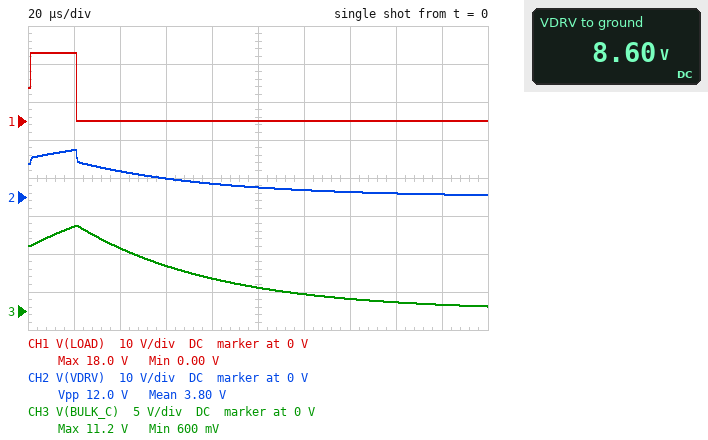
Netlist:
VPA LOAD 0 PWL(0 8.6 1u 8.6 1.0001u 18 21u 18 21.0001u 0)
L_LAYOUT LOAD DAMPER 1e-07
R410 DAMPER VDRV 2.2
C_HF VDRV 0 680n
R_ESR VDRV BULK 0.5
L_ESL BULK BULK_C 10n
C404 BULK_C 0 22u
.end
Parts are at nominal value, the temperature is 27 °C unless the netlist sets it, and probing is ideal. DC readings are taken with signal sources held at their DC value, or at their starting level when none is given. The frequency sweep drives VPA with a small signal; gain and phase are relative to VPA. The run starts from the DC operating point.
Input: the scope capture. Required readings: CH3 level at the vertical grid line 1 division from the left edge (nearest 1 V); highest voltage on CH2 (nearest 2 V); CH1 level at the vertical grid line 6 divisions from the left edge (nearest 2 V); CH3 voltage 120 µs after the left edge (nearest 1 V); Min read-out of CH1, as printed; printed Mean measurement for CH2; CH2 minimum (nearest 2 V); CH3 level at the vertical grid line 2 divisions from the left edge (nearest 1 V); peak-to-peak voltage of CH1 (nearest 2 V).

11 V
12 V
0 V
2 V
0.00 V
3.80 V
0 V
8 V
18 V
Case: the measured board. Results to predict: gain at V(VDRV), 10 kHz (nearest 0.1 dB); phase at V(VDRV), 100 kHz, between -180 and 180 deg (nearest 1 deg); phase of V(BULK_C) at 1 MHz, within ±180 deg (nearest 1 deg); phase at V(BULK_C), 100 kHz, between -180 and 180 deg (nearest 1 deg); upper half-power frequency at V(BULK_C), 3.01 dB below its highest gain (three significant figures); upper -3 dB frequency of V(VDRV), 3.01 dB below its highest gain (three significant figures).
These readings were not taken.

-10.2 dB
-17 deg
-171 deg
-100 deg
2.63 kHz
2.72 kHz
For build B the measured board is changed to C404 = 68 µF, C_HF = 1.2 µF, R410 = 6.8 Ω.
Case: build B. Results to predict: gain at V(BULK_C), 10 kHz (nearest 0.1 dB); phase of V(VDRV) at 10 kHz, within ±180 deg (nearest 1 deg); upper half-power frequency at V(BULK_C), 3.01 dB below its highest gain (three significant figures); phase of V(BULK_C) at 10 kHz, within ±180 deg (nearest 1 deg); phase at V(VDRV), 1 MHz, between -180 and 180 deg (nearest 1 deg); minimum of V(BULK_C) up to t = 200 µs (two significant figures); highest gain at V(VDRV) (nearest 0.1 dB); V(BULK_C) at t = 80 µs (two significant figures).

-30.0 dB
-25 deg
316 Hz
-90 deg
-79 deg
6.3 V
0 dB
8.0 V
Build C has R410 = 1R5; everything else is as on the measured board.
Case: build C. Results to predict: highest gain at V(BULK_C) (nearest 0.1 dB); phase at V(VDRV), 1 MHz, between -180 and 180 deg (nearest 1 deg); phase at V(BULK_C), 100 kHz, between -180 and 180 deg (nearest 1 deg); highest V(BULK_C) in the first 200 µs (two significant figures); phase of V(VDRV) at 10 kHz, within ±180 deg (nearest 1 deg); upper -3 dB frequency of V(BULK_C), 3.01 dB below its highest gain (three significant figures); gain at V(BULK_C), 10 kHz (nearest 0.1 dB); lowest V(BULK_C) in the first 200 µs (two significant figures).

0 dB
-79 deg
-99 deg
12 V
-37 deg
3.56 kHz
-9.5 dB
220 mV
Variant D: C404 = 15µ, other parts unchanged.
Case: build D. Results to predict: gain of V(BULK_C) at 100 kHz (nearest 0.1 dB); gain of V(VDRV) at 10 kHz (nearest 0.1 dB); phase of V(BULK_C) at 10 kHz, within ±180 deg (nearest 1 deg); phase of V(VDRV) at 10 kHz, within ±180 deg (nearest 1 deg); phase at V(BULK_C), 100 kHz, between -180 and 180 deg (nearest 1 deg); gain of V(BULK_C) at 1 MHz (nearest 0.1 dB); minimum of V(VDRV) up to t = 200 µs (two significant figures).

-28.5 dB
-8.1 dB
-70 deg
-45 deg
-99 deg
-54.0 dB
140 mV
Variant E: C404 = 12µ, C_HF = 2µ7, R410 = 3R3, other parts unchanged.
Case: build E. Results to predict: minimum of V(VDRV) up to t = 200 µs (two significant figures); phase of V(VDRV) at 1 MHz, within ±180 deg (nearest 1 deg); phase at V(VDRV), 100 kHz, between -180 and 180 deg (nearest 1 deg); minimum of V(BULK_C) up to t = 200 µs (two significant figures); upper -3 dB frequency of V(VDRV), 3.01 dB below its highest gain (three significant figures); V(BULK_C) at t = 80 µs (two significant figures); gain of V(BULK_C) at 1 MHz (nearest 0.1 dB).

370 mV
-93 deg
-46 deg
410 mV
3.01 kHz
3.9 V
-66.6 dB
